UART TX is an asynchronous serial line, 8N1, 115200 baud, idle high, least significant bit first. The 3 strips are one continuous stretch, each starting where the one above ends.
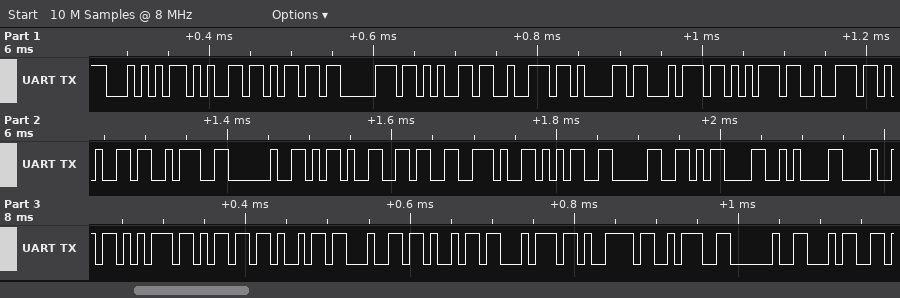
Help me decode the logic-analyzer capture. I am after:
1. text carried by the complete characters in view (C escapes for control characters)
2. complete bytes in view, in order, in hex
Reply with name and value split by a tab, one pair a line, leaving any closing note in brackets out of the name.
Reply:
text carried by the complete characters in view	"Temperature: -6.50\r\nHumidity: 4"
complete bytes in view, in order, in hex	54 65 6D 70 65 72 61 74 75 72 65 3A 20 2D 36 2E 35 30 0D 0A 48 75 6D 69 64 69 74 79 3A 20 34
